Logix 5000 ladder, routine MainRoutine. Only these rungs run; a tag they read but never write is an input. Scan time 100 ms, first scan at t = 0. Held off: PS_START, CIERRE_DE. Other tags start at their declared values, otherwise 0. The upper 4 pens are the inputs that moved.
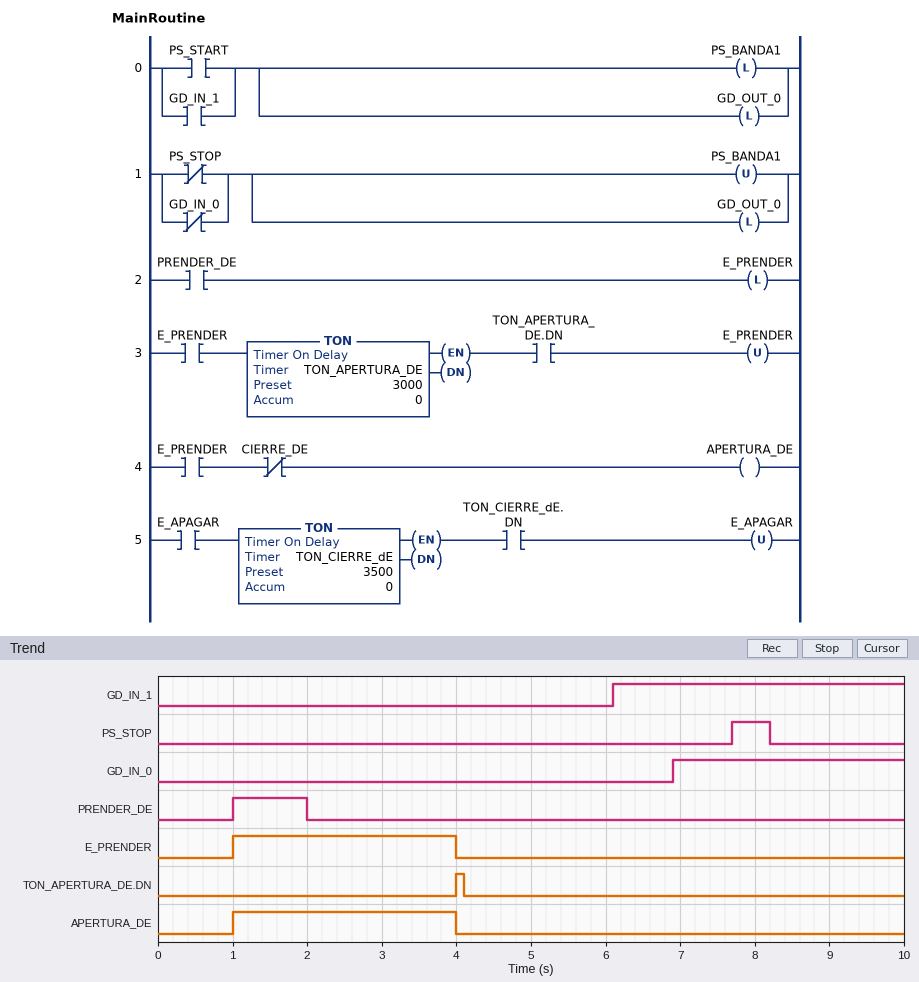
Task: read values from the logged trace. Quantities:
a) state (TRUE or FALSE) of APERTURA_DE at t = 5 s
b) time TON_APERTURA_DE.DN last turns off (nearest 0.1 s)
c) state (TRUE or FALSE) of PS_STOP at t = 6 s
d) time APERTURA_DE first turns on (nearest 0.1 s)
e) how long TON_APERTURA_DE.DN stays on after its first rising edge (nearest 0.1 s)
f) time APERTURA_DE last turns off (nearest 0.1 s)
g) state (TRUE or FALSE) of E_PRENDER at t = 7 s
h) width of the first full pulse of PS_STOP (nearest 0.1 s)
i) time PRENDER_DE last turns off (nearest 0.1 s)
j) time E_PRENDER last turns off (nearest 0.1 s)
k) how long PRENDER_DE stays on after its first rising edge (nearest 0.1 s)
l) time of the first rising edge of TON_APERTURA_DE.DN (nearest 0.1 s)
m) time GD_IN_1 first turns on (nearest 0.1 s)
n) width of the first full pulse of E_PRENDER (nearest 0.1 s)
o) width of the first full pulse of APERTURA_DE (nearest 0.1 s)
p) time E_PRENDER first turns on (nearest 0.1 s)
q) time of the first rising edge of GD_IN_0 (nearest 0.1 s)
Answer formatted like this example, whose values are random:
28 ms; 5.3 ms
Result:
FALSE; 4.1 s; FALSE; 1.0 s; 0.1 s; 4.0 s; FALSE; 0.5 s; 2.0 s; 4.0 s; 1.0 s; 4.0 s; 6.1 s; 3.0 s; 3.0 s; 1.0 s; 6.9 s
